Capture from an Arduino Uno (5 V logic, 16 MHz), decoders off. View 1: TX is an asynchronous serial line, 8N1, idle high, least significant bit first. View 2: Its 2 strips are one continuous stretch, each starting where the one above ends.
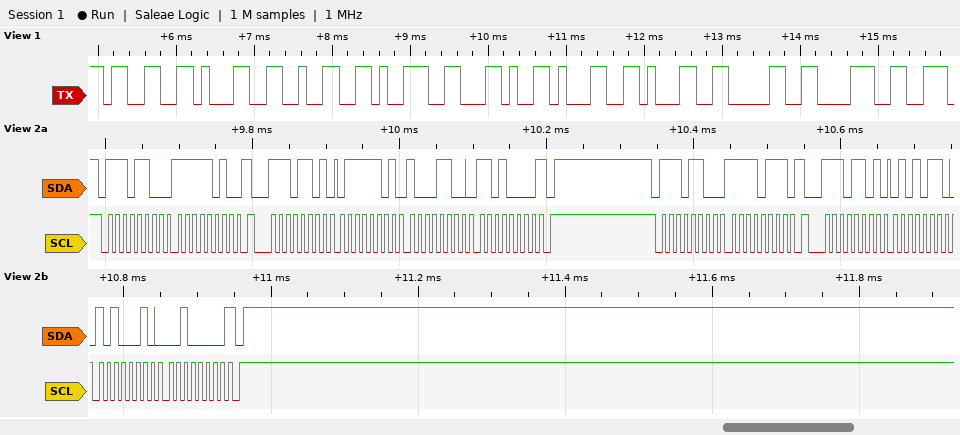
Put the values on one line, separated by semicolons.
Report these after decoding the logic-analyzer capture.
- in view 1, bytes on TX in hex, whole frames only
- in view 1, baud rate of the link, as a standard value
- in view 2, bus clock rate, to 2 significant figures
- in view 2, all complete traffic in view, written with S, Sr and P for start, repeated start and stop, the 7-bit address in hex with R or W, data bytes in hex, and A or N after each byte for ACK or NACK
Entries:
33 31 32 39 2C 31 31 30 38; 9600 baud; 100 kHz; S 76W A FA A Sr 76R A 7D A 8C A D0 N P S 76W A F7 A Sr 76R A 56 A A2 A 20 N P
